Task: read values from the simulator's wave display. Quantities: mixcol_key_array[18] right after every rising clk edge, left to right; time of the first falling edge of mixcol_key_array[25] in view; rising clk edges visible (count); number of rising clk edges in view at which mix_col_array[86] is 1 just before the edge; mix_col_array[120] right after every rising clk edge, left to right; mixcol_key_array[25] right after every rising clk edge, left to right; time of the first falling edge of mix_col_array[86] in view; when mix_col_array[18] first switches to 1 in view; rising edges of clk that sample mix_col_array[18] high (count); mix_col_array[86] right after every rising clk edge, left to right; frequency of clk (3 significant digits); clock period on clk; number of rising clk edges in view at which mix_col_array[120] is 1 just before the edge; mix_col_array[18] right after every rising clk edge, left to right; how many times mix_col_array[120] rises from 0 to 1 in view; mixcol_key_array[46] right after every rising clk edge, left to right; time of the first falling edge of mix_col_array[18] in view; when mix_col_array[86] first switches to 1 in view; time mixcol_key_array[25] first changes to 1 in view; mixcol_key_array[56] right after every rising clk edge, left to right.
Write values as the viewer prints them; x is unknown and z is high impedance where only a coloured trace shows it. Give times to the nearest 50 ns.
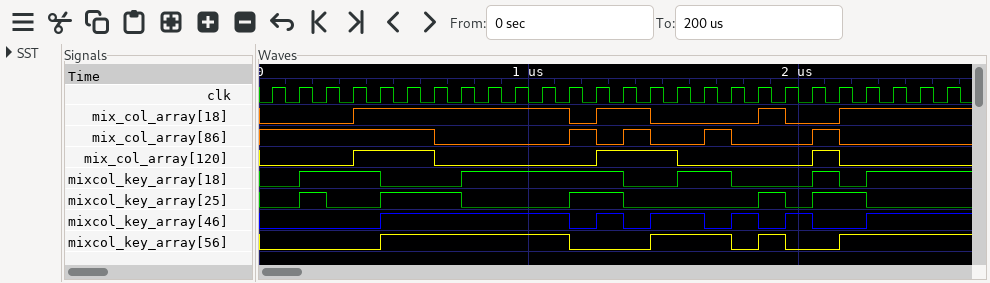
0 1 1 1 0 0 0 1 1 1 1 1 1 0 0 1 1 0 0 0 1 0 1 1 1 1
250 ns
26
11
0 0 0 1 1 1 0 0 0 0 0 0 1 1 1 0 0 0 0 0 1 0 0 0 0 0
0 1 0 0 1 1 1 0 0 0 0 1 1 0 0 0 0 0 1 0 1 1 0 0 0 0
650 ns
350 ns
15
1 1 1 1 1 1 0 0 0 0 0 1 0 1 0 0 1 0 0 0 1 0 0 0 0 0
10.0 MHz
100 ns
7
0 0 0 1 1 1 1 1 1 1 1 0 1 1 0 0 0 0 1 0 0 1 1 1 1 1
3
0 0 0 0 1 1 1 1 1 1 1 0 1 0 1 1 0 1 0 1 0 0 1 1 1 1
1150 ns
1150 ns
150 ns
0 0 0 0 1 1 1 1 1 1 1 0 0 0 1 1 1 0 1 0 0 1 1 1 1 1
